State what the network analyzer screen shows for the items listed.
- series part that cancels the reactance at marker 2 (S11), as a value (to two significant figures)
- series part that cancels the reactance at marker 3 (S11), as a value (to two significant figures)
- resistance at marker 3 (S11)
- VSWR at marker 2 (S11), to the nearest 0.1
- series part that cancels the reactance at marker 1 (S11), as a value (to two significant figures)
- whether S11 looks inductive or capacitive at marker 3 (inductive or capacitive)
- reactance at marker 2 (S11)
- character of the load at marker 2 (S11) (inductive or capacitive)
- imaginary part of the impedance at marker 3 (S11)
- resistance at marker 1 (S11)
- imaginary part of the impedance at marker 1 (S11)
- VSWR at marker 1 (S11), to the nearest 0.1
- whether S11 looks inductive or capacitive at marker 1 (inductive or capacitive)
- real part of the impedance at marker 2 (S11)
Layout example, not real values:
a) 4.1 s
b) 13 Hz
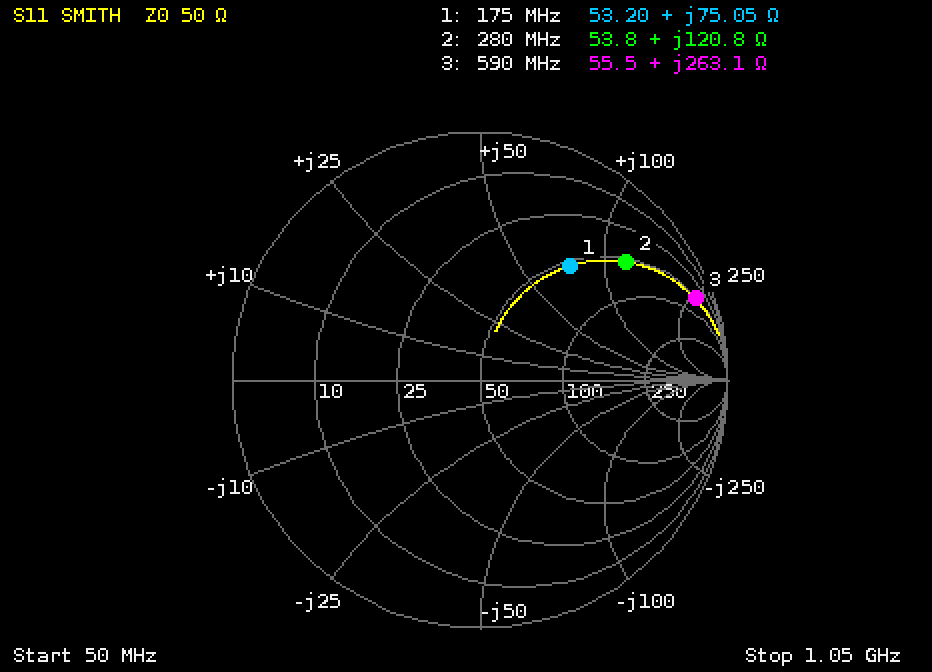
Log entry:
a) 4.7 pF
b) 1.0 pF
c) 55.5 Ω
d) 7.3
e) 12 pF
f) inductive
g) +120.8 Ω
h) inductive
i) +263.1 Ω
j) 53.20 Ω
k) +75.05 Ω
l) 3.9
m) inductive
n) 53.8 Ω
